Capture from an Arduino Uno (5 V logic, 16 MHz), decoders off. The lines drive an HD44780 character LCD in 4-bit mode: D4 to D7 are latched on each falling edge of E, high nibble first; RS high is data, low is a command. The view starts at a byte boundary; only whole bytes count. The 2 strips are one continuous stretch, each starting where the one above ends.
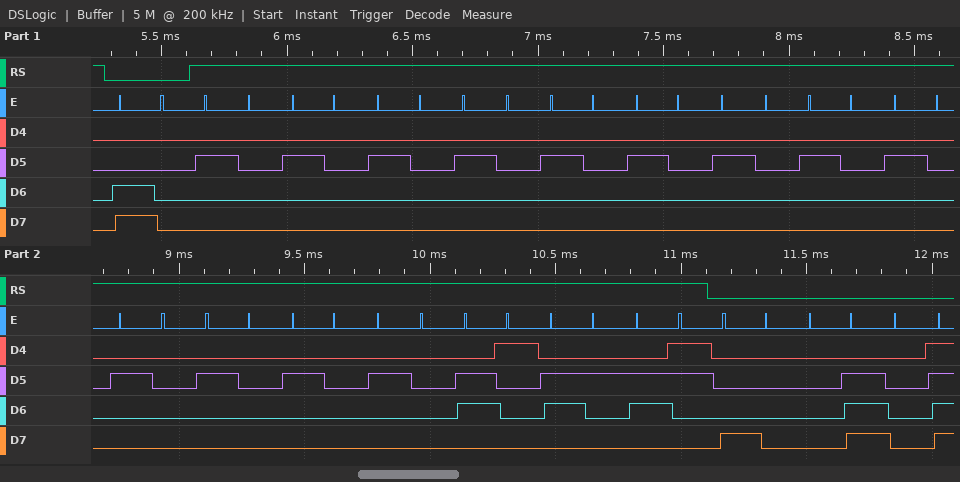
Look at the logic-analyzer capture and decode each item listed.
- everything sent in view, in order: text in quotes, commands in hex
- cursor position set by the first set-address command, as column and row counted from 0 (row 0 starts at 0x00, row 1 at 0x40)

0xC0 "             abc" 0x80 0x0E 0x0F
column 0, row 1
